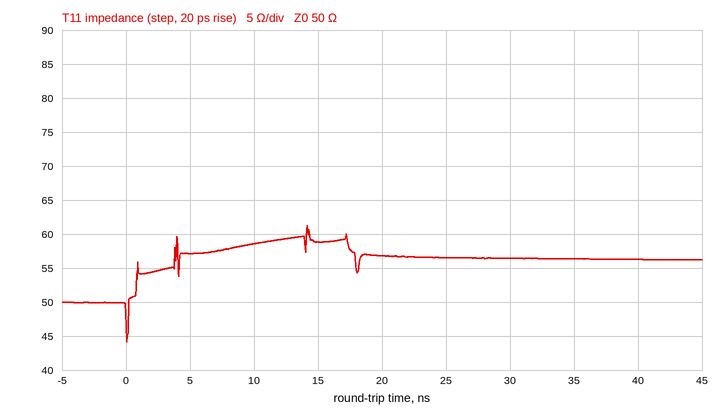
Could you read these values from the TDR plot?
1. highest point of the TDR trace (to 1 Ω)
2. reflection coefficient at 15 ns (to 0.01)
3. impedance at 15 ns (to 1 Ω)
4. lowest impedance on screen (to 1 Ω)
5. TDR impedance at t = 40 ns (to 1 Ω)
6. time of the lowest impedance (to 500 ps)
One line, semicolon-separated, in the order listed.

61 Ω; +0.08; 59 Ω; 44 Ω; 56 Ω; 0.0 ns
